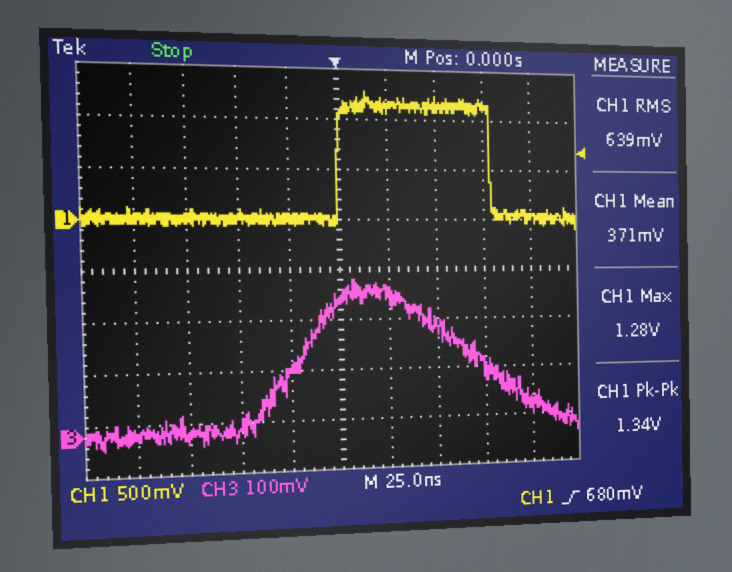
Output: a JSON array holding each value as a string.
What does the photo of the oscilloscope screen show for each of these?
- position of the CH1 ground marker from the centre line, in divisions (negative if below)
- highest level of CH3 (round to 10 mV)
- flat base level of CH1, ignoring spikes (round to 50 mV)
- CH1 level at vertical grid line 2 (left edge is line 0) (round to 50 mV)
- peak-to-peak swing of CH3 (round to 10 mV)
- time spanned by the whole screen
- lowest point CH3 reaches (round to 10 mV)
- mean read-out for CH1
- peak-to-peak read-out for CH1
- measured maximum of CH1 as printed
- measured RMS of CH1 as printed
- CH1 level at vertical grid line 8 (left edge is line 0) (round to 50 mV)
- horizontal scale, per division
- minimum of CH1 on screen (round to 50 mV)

["+1.0 div", "300 mV", "0 mV", "0 mV", "330 mV", "250 ns", "-30 mV", "371 mV", "1.34 V", "1.28 V", "639 mV", "1.15 V", "25 ns", "-100 mV"]
